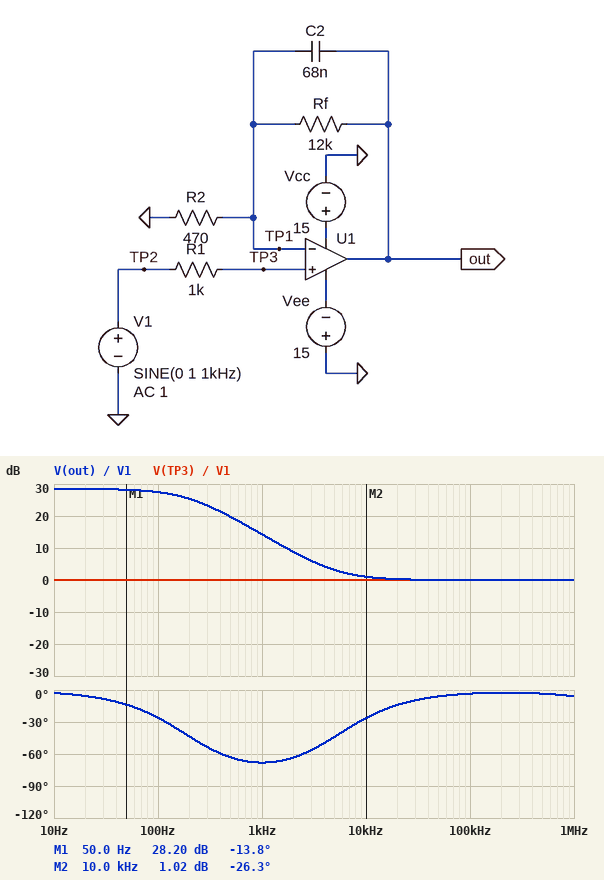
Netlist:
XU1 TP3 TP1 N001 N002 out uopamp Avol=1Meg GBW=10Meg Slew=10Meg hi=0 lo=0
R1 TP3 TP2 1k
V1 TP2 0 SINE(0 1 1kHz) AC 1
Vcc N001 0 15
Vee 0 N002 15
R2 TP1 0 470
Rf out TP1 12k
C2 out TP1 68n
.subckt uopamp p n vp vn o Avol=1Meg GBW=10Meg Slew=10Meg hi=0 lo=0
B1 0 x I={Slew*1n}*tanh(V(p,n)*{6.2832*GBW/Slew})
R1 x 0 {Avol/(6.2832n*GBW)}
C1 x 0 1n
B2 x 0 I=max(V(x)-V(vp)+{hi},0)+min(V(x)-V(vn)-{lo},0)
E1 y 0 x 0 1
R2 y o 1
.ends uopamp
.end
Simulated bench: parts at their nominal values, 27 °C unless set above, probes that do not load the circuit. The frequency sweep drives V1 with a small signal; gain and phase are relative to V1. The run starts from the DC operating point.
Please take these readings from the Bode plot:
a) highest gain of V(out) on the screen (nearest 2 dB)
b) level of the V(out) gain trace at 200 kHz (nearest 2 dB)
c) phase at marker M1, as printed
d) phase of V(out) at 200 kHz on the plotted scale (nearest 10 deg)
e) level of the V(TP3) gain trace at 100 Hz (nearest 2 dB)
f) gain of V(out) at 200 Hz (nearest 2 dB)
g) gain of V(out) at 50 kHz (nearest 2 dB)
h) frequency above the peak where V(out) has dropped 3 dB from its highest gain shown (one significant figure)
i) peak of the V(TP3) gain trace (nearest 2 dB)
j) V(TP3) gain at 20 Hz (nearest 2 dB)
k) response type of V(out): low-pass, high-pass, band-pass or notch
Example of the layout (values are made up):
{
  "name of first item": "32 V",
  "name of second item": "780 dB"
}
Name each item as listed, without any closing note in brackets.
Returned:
{
  "highest gain of V(out) on the screen": "28 dB",
  "level of the V(out) gain trace at 200 kHz": "0 dB",
  "phase at marker M1, as printed": "-13.8 deg",
  "phase of V(out) at 200 kHz on the plotted scale": "0 deg",
  "level of the V(TP3) gain trace at 100 Hz": "0 dB",
  "gain of V(out) at 200 Hz": "26 dB",
  "gain of V(out) at 50 kHz": "0 dB",
  "frequency above the peak where V(out) has dropped 3 dB from its highest gain shown": "200 Hz",
  "peak of the V(TP3) gain trace": "0 dB",
  "V(TP3) gain at 20 Hz": "0 dB",
  "response type of V(out): low-pass, high-pass, band-pass or notch": "low-pass"
}
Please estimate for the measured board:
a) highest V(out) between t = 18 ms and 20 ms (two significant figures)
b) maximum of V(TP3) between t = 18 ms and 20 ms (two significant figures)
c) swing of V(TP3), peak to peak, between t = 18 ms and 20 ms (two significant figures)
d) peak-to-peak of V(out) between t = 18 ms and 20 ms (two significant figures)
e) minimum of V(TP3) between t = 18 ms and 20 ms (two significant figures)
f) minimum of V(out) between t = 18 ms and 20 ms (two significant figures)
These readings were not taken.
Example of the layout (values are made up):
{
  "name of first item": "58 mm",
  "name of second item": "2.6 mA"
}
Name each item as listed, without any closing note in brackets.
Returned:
{
  "highest V(out) between t = 18 ms and 20 ms": "5.2 V",
  "maximum of V(TP3) between t = 18 ms and 20 ms": "1.0 V",
  "swing of V(TP3), peak to peak, between t = 18 ms and 20 ms": "2.0 V",
  "peak-to-peak of V(out) between t = 18 ms and 20 ms": "10 V",
  "minimum of V(TP3) between t = 18 ms and 20 ms": "-1.0 V",
  "minimum of V(out) between t = 18 ms and 20 ms": "-5.2 V"
}
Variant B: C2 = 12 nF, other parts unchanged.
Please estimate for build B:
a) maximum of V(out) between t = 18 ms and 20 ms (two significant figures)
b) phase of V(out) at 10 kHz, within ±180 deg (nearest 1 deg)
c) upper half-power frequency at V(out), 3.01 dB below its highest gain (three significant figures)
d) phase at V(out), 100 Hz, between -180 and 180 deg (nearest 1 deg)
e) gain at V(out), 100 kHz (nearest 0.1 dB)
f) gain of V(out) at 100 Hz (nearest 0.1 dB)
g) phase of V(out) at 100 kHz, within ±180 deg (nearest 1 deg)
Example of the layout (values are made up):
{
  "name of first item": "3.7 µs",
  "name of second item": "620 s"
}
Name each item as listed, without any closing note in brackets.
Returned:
{
  "maximum of V(out) between t = 18 ms and 20 ms": "15 V",
  "phase of V(out) at 10 kHz, within ±180 deg": "-65 deg",
  "upper half-power frequency at V(out), 3.01 dB below its highest gain": "1.10 kHz",
  "phase at V(out), 100 Hz, between -180 and 180 deg": "-5 deg",
  "gain at V(out), 100 kHz": "0.3 dB",
  "gain of V(out) at 100 Hz": "28.4 dB",
  "phase of V(out) at 100 kHz, within ±180 deg": "-16 deg"
}
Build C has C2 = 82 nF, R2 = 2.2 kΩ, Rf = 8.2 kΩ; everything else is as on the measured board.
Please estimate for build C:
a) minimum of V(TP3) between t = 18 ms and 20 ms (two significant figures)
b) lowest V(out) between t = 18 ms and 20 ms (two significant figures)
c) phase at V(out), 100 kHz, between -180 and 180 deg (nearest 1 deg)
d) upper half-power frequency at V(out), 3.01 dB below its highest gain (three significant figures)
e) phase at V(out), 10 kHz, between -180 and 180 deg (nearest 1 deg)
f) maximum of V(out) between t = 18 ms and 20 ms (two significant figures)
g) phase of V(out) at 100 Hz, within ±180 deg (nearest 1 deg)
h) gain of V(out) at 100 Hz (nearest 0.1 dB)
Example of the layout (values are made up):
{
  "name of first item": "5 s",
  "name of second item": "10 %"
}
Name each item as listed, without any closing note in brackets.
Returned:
{
  "minimum of V(TP3) between t = 18 ms and 20 ms": "-1.0 V",
  "lowest V(out) between t = 18 ms and 20 ms": "-1.5 V",
  "phase at V(out), 100 kHz, between -180 and 180 deg": "-1 deg",
  "upper half-power frequency at V(out), 3.01 dB below its highest gain": "248 Hz",
  "phase at V(out), 10 kHz, between -180 and 180 deg": "-5 deg",
  "maximum of V(out) between t = 18 ms and 20 ms": "1.5 V",
  "phase of V(out) at 100 Hz, within ±180 deg": "-18 deg",
  "gain of V(out) at 100 Hz": "12.8 dB"
}
